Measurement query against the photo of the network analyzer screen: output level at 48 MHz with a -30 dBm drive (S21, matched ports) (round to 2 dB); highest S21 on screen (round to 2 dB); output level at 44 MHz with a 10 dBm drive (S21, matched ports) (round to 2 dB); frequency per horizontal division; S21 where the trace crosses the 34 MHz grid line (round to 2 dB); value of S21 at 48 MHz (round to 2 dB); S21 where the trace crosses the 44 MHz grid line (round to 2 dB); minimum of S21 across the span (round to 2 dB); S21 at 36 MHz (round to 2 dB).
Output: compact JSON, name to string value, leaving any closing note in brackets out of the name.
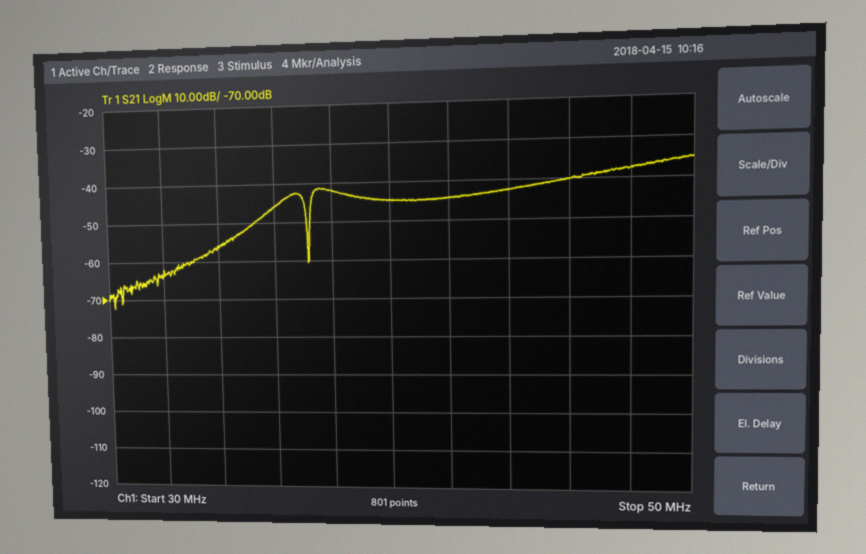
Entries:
{"output level at 48 MHz with a -30 dBm drive (S21, matched ports)": "-68 dBm", "highest S21 on screen": "-36 dB", "output level at 44 MHz with a 10 dBm drive (S21, matched ports)": "-32 dBm", "frequency per horizontal division": "2 MHz", "S21 where the trace crosses the 34 MHz grid line": "-56 dB", "value of S21 at 48 MHz": "-38 dB", "S21 where the trace crosses the 44 MHz grid line": "-42 dB", "minimum of S21 across the span": "-72 dB", "S21 at 36 MHz": "-46 dB"}
